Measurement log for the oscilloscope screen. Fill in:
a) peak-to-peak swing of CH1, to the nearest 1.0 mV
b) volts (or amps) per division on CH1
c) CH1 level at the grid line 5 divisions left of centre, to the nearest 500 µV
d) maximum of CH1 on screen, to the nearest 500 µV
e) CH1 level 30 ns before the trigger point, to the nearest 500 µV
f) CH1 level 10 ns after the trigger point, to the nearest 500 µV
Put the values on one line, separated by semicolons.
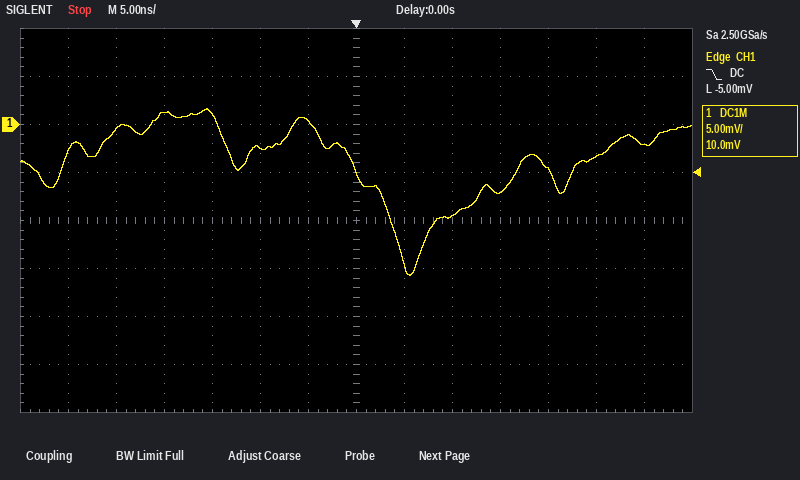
17.0 mV; 5 mV; -500 µV; 1.5 mV; -3.0 mV; -9.5 mV
